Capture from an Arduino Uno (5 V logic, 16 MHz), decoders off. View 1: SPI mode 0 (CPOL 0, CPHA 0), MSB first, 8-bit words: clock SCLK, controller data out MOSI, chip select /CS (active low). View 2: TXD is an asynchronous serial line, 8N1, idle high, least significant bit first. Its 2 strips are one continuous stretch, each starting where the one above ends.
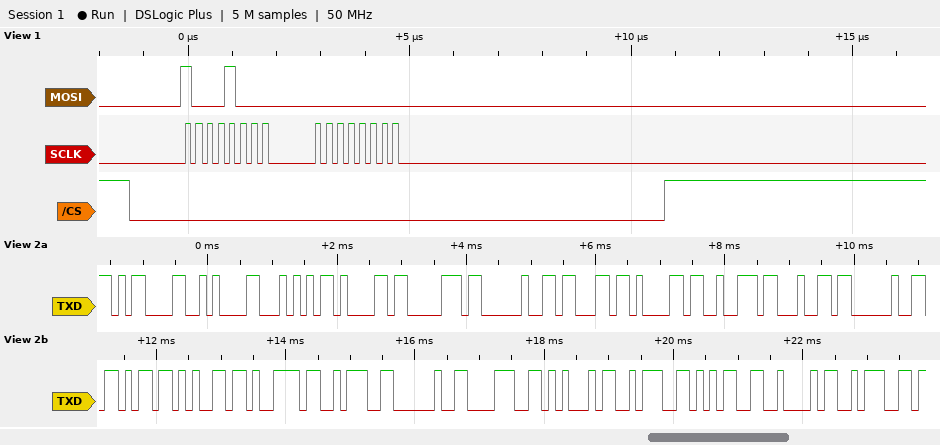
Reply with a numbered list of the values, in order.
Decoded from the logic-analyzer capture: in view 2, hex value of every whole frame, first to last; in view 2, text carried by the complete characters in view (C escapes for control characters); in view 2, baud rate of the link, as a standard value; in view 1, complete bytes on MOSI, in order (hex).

1. 0x0D 0x0A 0x54 0x61 0x70 0x20 0x63 0x61 0x72 0x64 0x20 0x6B 0x65 0x79 0x3A 0x20 0x38 0x45 0x3A 0x35 0x42 0x3A
2. "\r\nTap card key: 8E:5B:"
3. 9600 baud
4. 0x88 0x00
